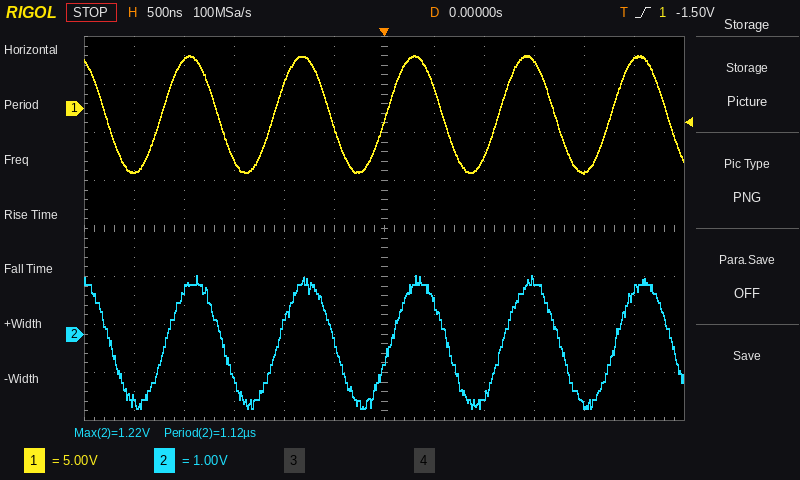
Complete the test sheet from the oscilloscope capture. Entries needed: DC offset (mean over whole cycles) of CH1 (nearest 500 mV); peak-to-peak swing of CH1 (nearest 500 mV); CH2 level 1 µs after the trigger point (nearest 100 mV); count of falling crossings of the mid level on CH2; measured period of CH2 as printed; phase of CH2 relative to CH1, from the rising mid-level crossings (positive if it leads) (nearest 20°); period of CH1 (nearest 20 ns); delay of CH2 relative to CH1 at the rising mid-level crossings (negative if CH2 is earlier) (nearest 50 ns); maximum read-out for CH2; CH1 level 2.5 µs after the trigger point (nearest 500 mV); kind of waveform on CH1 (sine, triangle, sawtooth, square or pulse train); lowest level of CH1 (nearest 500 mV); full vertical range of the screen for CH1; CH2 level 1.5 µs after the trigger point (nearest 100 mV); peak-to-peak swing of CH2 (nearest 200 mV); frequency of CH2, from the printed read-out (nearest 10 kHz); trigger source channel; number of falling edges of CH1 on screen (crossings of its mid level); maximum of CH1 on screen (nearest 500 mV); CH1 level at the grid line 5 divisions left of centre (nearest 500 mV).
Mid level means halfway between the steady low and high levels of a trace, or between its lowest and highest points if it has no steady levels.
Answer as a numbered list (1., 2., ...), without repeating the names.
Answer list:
1. -500 mV
2. 12.5 V
3. -1.3 V
4. 6
5. 1.12 µs
6. -20°
7. 1.12 µs
8. +50 ns
9. 1.22 V
10. 5.0 V
11. sine
12. -7.0 V
13. 40 V
14. 1.1 V
15. 2.8 V
16. 890 kHz
17. CH1
18. 6
19. 5.5 V
20. -6.5 V
